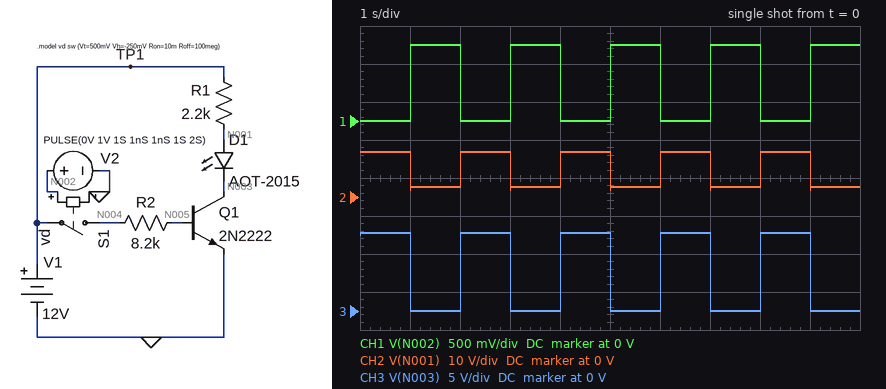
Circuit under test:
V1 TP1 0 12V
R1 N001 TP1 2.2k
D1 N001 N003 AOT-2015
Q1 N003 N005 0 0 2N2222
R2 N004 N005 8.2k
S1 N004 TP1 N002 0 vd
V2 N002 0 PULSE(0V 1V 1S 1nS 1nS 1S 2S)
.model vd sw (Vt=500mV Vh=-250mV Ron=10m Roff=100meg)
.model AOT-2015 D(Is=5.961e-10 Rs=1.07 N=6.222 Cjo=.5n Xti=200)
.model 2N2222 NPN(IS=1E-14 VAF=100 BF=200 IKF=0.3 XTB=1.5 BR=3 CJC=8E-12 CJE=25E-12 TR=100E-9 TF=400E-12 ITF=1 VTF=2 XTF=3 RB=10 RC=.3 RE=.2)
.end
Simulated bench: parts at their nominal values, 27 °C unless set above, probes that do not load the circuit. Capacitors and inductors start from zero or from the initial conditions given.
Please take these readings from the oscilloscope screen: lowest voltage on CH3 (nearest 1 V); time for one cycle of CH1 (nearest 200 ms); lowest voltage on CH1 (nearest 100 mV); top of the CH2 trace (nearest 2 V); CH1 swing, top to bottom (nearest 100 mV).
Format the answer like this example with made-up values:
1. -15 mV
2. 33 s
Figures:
1. 0 V
2. 2.0 s
3. 0 V
4. 12 V
5. 1.0 V
